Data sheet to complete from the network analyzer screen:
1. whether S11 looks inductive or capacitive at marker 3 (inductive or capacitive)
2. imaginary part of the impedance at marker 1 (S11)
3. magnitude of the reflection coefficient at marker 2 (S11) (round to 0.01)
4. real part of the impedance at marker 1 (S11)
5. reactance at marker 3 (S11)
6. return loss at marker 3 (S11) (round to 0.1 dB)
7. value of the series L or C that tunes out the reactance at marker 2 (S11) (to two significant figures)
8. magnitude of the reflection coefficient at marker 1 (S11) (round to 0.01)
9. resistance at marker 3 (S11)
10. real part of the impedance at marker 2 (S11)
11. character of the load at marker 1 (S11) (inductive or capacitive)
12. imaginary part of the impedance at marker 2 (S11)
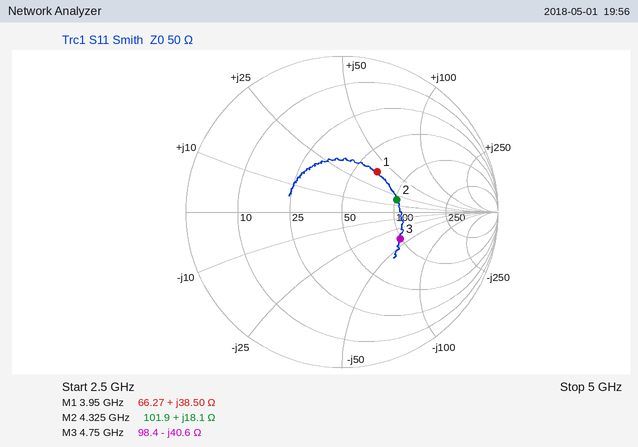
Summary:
capacitive
+38.50 Ω
0.36
66.27 Ω
-40.6 Ω
7.7 dB
2.0 pF
0.34
98.4 Ω
101.9 Ω
inductive
+18.1 Ω
